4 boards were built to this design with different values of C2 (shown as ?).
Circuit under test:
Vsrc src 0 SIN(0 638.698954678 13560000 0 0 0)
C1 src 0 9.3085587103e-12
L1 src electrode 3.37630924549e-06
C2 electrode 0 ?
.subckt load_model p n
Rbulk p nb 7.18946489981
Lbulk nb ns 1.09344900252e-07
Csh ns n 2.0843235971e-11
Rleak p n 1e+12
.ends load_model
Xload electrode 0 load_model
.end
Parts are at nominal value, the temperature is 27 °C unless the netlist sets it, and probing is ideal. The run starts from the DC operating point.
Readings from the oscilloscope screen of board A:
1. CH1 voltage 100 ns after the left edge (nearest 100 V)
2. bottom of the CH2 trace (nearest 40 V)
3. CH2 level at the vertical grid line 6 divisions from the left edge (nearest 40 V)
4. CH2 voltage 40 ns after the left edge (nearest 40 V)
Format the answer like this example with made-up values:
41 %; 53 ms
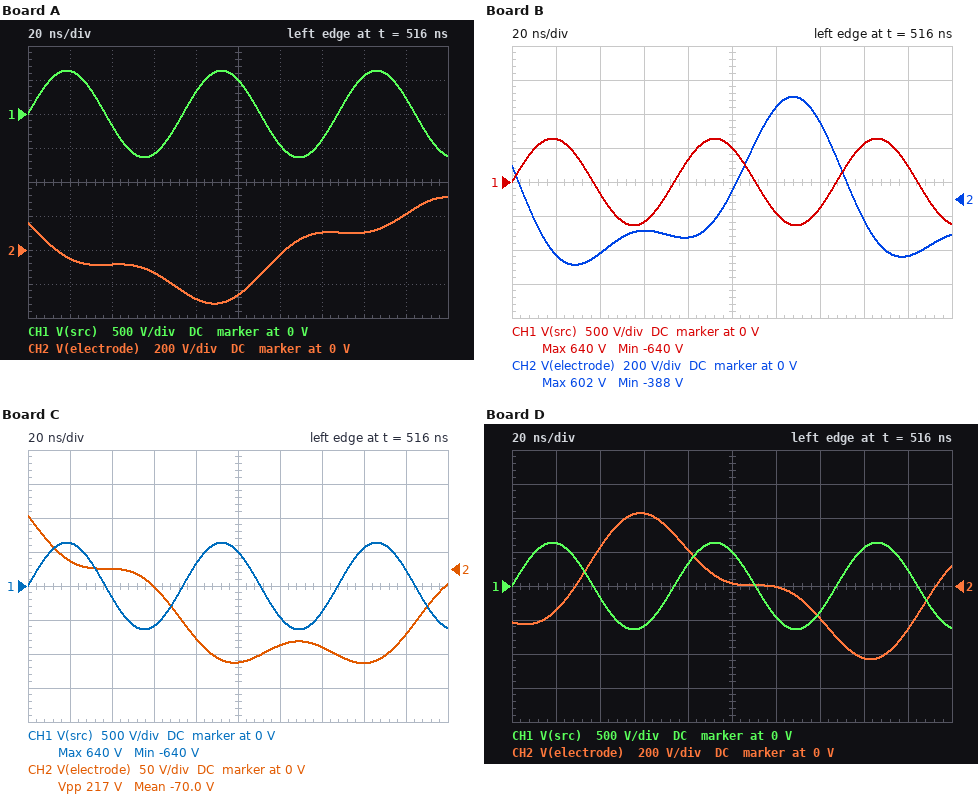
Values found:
500 V; -320 V; -40 V; -80 V
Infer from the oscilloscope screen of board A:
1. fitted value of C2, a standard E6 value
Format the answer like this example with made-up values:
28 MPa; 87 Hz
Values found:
330 pF
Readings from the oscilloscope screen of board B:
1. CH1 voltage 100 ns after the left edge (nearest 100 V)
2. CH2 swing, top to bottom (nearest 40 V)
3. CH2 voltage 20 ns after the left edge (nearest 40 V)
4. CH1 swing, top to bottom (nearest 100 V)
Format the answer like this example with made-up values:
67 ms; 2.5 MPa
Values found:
500 V; 1.00 kV; -320 V; 1.3 kV
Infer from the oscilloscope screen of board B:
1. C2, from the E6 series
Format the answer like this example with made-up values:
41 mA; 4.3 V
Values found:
150 pF
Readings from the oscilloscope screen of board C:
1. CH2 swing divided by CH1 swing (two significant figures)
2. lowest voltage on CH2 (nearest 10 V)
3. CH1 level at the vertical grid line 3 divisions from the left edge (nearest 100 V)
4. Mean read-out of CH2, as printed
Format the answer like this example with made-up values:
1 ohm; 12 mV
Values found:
0.17; -140 V; -600 V; -70.0 V
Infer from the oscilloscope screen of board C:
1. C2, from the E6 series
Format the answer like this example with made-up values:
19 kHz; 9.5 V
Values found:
1 nF
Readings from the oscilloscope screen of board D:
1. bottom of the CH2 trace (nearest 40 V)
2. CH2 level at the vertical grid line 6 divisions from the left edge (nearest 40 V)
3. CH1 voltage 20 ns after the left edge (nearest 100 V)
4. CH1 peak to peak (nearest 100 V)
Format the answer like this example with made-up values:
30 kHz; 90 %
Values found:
-440 V; 0 V; 600 V; 1.3 kV
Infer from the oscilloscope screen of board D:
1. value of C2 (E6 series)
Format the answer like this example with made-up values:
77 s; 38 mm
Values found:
220 pF
